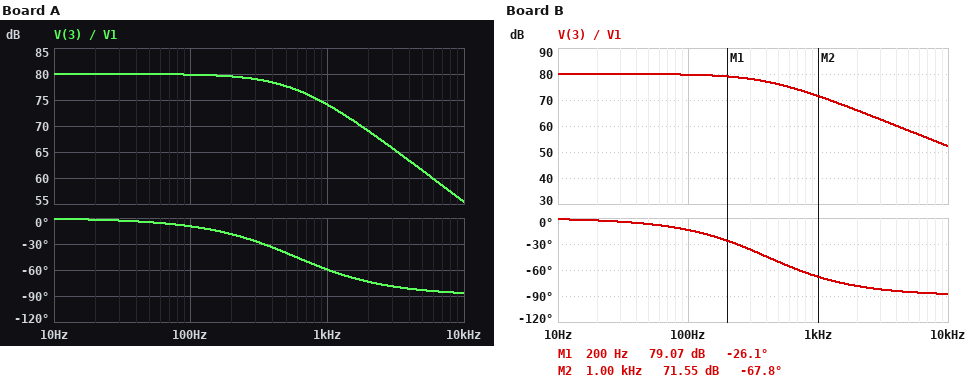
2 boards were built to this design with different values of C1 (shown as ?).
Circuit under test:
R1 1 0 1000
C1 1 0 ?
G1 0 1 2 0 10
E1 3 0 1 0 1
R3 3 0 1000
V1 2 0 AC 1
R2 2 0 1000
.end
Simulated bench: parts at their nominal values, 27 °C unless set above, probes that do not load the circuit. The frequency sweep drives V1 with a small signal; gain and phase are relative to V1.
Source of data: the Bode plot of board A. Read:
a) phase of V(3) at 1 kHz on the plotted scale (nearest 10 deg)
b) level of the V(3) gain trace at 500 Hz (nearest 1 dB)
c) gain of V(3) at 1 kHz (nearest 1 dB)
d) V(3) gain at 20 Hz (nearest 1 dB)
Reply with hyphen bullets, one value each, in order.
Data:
- -60 deg
- 78 dB
- 74 dB
- 80 dB
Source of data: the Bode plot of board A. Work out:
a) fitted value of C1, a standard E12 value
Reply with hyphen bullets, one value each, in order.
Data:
- 270 nF
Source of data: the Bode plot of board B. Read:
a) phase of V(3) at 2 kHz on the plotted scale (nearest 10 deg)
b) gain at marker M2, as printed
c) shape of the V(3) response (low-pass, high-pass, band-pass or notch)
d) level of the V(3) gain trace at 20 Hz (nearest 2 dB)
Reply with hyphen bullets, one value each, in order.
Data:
- -80 deg
- 71.55 dB
- low-pass
- 80 dB
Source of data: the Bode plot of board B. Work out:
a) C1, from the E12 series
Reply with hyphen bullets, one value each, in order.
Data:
- 390 nF
